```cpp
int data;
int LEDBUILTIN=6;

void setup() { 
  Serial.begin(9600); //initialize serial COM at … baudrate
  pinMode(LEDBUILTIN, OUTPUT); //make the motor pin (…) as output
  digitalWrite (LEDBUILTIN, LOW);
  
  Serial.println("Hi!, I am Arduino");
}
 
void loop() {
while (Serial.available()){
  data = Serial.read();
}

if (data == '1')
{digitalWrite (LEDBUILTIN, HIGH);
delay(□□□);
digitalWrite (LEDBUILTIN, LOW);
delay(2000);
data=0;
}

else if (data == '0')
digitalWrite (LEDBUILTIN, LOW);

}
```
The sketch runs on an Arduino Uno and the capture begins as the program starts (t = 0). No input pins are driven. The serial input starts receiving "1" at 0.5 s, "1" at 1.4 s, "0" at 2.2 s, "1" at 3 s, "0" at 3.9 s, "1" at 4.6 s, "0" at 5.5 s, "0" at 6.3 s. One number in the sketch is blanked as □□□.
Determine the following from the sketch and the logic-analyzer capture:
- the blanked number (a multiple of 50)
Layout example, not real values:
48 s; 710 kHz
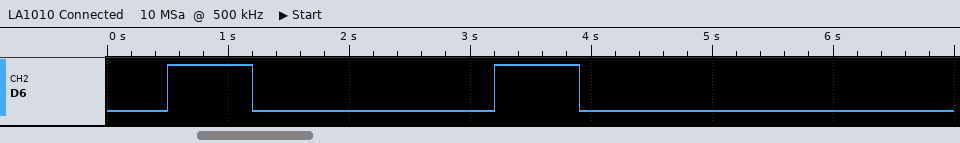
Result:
700
